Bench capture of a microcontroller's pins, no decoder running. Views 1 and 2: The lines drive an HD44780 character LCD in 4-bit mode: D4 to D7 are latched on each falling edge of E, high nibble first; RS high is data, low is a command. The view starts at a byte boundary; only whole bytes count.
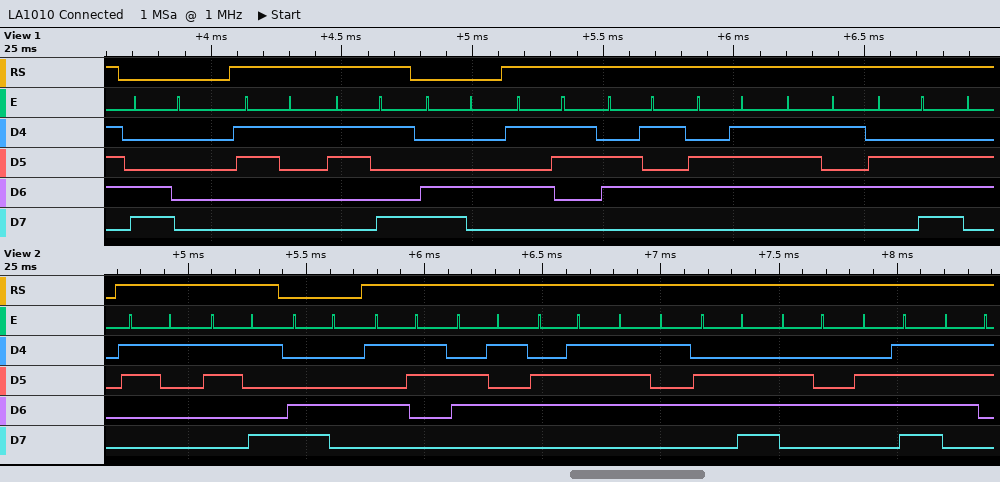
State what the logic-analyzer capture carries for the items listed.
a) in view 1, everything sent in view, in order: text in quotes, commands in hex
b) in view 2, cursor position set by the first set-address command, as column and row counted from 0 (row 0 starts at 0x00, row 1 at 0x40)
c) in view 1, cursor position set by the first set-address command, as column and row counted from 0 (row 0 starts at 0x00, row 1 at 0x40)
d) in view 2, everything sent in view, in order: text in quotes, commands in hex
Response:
0xC0 "19" 0xC4 "Segun"
column 4, row 1
column 0, row 1
"19" 0xC4 "Segundos"
